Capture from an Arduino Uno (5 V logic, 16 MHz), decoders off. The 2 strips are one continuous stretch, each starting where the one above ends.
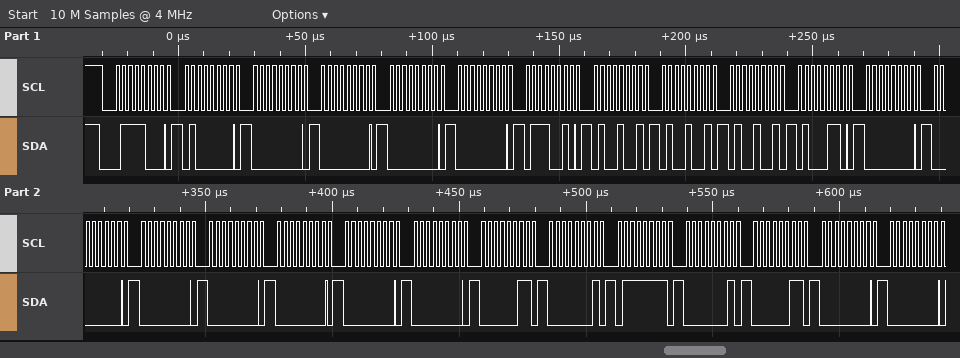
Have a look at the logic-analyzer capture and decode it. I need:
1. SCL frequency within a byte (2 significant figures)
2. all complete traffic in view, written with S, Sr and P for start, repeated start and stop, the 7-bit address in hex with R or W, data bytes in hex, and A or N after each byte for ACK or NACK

400 kHz
S 3CW A 40 A 00 A 00 A 00 A 00 A 72 A 49 A 49 A 49 A 46 A 00 A 00 A 00 A 00 A 00 A 00 A 00 A 03 A 01 A 7F A 01 A 03 A 00 A 00 A
